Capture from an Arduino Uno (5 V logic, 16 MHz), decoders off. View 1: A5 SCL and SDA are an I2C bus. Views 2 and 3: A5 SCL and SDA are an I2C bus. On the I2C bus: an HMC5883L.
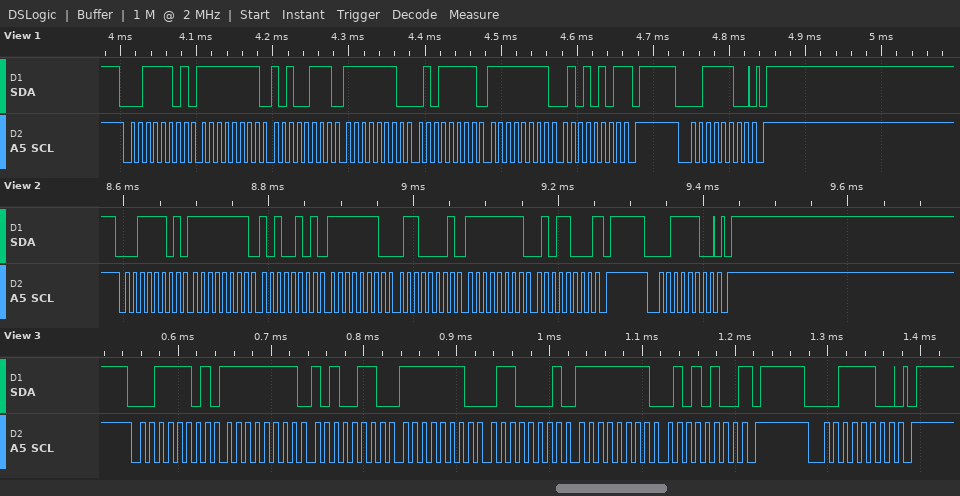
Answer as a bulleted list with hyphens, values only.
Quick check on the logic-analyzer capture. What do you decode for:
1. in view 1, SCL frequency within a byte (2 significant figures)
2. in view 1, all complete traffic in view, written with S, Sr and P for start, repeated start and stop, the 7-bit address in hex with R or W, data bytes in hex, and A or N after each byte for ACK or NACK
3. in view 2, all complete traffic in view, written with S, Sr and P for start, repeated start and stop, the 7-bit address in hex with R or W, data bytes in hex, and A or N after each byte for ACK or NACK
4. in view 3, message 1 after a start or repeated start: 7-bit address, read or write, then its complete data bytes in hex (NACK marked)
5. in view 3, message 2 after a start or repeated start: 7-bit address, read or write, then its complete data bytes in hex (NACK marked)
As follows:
- 100 kHz
- S 1ER A FF A A7 A FE A 5F A FF A 55 N P S 1EW A P
- S 1ER A FF A A5 A FE A 61 A FF A 58 N P S 1EW A P
- 0x1E read: FF A6 FE 61 FF 54 NACK
- 0x1E write
